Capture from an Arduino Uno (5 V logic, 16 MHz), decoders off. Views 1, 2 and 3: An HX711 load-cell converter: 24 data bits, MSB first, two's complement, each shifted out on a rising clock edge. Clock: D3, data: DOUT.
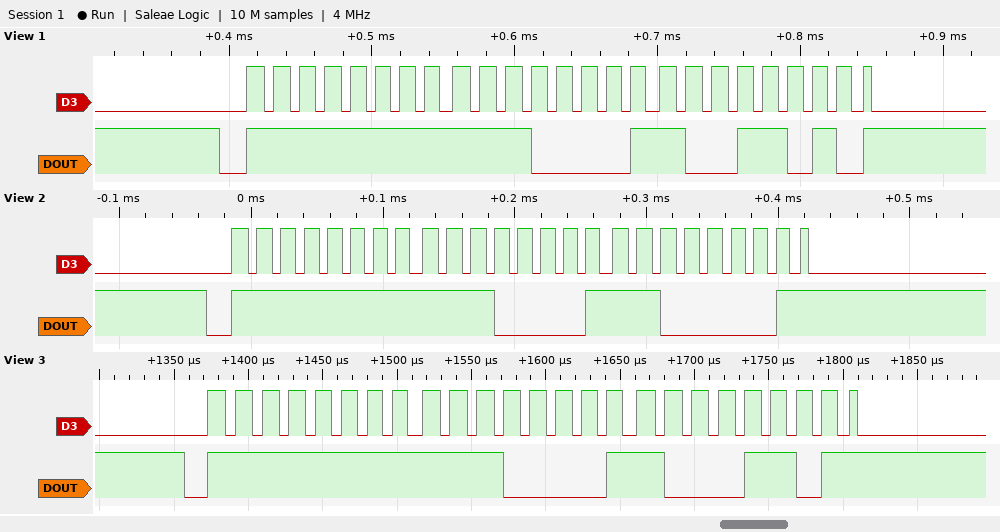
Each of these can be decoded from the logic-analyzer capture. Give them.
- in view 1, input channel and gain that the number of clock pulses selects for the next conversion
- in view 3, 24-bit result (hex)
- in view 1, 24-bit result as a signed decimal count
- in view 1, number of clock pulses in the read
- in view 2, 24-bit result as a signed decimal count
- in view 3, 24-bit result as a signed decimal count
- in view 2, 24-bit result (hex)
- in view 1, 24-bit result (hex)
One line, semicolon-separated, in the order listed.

channel A, gain 128; 0xFFE18D; -7782; 25; -7743; -7795; 0xFFE1C1; 0xFFE19A
